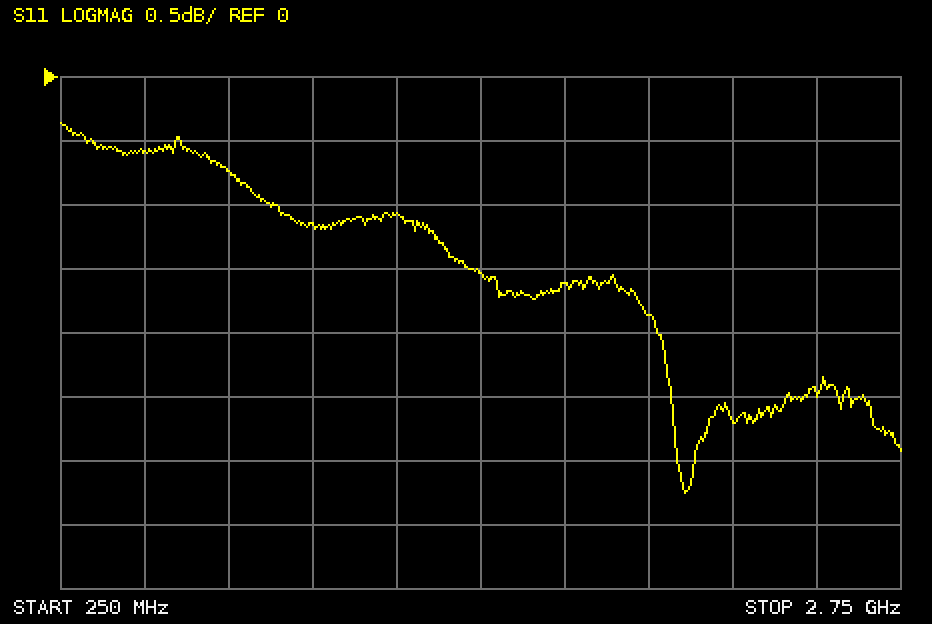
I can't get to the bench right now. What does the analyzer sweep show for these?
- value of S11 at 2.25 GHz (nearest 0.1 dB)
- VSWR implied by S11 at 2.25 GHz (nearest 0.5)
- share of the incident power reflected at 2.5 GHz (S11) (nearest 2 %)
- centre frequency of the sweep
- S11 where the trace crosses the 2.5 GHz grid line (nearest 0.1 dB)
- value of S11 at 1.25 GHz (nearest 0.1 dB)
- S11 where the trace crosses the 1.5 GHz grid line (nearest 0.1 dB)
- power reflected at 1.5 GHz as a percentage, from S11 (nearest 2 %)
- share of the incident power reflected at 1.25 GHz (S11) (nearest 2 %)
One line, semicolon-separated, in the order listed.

-2.7 dB; 6.5; 56 %; 1.5 GHz; -2.5 dB; -1.1 dB; -1.5 dB; 70 %; 78 %
